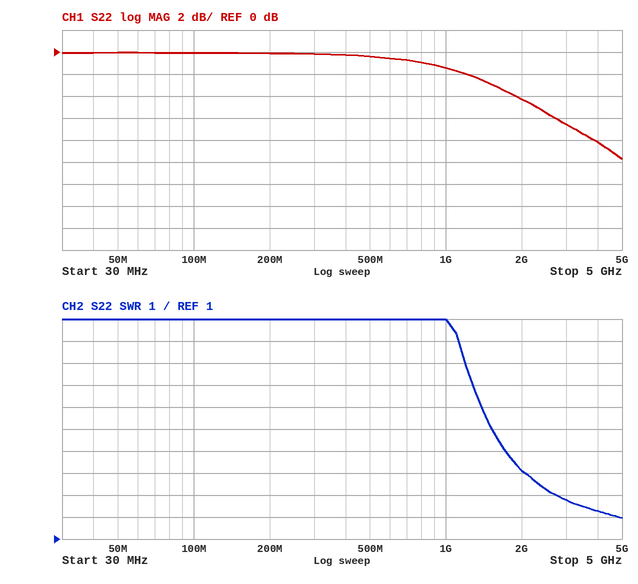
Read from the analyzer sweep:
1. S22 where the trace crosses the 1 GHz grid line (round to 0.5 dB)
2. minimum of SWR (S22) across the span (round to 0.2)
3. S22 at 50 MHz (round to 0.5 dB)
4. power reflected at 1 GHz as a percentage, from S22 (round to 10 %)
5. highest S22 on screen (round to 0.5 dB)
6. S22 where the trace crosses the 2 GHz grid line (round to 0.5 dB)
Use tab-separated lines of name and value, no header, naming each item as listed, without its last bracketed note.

S22 where the trace crosses the 1 GHz grid line	-1.5 dB
minimum of SWR (S22) across the span	2.0
S22 at 50 MHz	0.0 dB
power reflected at 1 GHz as a percentage, from S22	70 %
highest S22 on screen	0.0 dB
S22 where the trace crosses the 2 GHz grid line	-4.5 dB
